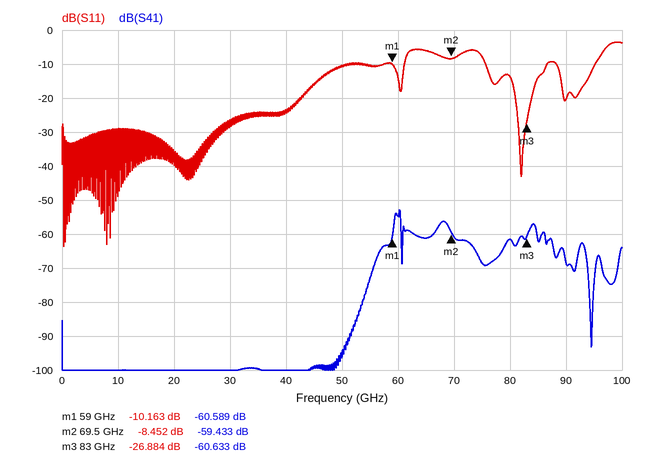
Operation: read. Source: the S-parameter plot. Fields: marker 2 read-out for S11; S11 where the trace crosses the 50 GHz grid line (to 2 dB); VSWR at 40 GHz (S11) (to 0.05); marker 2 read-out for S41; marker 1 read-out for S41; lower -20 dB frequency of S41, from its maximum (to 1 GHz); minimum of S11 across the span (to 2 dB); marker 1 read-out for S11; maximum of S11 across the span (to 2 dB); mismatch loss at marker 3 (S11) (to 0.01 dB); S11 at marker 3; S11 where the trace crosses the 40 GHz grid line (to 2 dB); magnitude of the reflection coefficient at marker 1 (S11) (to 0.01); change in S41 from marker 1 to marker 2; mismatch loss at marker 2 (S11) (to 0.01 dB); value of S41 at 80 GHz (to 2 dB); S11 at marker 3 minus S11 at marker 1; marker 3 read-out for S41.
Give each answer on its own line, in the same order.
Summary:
-8.452 dB
-10 dB
1.15
-59.433 dB
-60.589 dB
55 GHz
-64 dB
-10.163 dB
-4 dB
0.01 dB
-26.884 dB
-24 dB
0.31
1.156 dB
0.67 dB
-62 dB
-16.721 dB
-60.633 dB
